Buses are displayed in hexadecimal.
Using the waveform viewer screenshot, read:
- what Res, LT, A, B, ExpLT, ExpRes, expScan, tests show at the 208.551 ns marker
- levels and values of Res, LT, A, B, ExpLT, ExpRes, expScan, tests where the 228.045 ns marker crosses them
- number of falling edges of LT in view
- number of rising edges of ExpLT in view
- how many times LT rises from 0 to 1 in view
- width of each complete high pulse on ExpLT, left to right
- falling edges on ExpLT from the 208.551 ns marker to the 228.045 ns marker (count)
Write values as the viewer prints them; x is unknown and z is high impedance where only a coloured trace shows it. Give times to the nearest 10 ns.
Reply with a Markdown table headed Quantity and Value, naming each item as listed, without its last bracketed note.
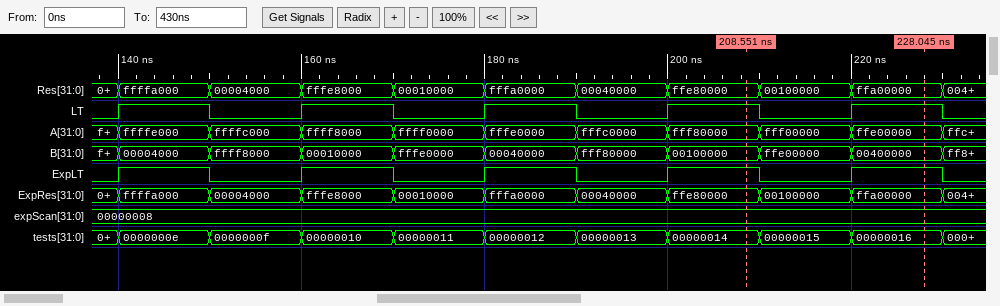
| Quantity | Value |
|---|---|
| what Res, LT, A, B, ExpLT, ExpRes, expScan, tests show at the 208.551 ns marker | Res=ffe80000, LT=1, A=fff80000, B=00100000, ExpLT=1, ExpRes=ffe80000, expScan=00000008, tests=00000014 |
| levels and values of Res, LT, A, B, ExpLT, ExpRes, expScan, tests where the 228.045 ns marker crosses them | Res=ffa00000, LT=1, A=ffe00000, B=00400000, ExpLT=1, ExpRes=ffa00000, expScan=00000008, tests=00000016 |
| number of falling edges of LT in view | 5 |
| number of rising edges of ExpLT in view | 5 |
| how many times LT rises from 0 to 1 in view | 5 |
| width of each complete high pulse on ExpLT, left to right | 10 ns, 10 ns, 10 ns, 10 ns, 10 ns |
| falling edges on ExpLT from the 208.551 ns marker to the 228.045 ns marker | 1 |
